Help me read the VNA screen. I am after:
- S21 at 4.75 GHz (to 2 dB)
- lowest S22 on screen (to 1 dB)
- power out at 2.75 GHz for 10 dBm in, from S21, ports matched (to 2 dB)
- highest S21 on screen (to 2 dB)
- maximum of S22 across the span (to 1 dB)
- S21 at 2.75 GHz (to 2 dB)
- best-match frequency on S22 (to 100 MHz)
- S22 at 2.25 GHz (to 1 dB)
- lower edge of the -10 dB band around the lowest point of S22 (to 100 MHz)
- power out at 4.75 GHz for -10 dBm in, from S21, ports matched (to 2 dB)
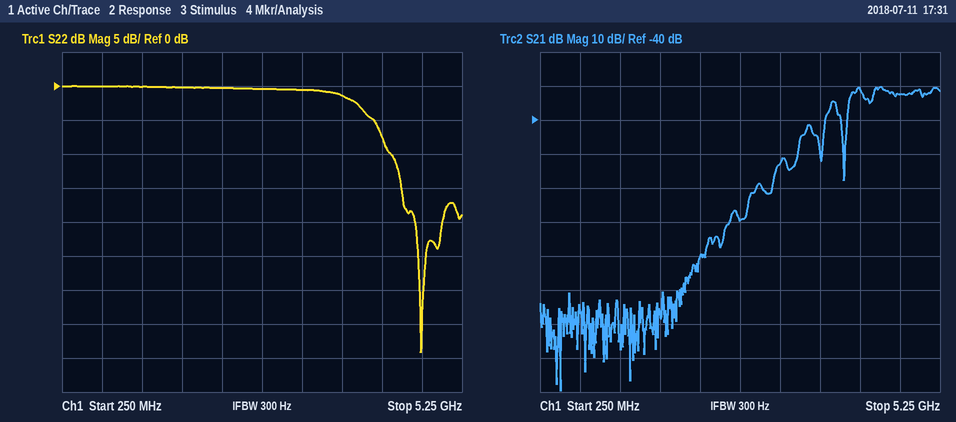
-32 dB
-39 dB
-60 dBm
-30 dB
0 dB
-70 dB
4.7 GHz
0 dB
4.4 GHz
-42 dBm
